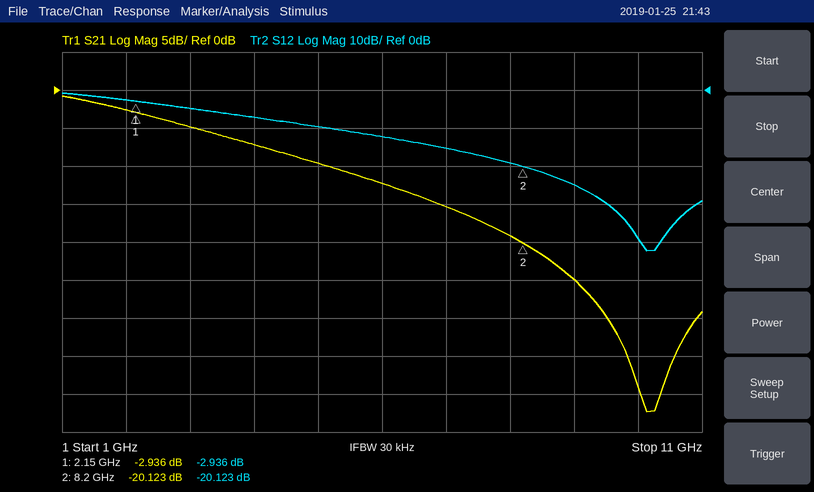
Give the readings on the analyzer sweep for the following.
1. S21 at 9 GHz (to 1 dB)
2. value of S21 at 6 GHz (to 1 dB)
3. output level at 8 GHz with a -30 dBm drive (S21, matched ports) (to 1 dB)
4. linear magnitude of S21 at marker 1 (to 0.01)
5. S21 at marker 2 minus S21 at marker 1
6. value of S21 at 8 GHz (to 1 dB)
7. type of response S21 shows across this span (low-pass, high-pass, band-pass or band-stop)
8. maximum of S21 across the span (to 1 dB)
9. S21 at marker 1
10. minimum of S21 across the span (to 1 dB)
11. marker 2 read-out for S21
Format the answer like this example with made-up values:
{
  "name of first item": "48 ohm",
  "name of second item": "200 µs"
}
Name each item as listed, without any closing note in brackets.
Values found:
{
  "S21 at 9 GHz": "-25 dB",
  "value of S21 at 6 GHz": "-12 dB",
  "output level at 8 GHz with a -30 dBm drive (S21, matched ports)": "-49 dBm",
  "linear magnitude of S21 at marker 1": "0.71",
  "S21 at marker 2 minus S21 at marker 1": "-17.187 dB",
  "value of S21 at 8 GHz": "-19 dB",
  "type of response S21 shows across this span": "low-pass",
  "maximum of S21 across the span": "-1 dB",
  "S21 at marker 1": "-2.936 dB",
  "minimum of S21 across the span": "-42 dB",
  "marker 2 read-out for S21": "-20.123 dB"
}
